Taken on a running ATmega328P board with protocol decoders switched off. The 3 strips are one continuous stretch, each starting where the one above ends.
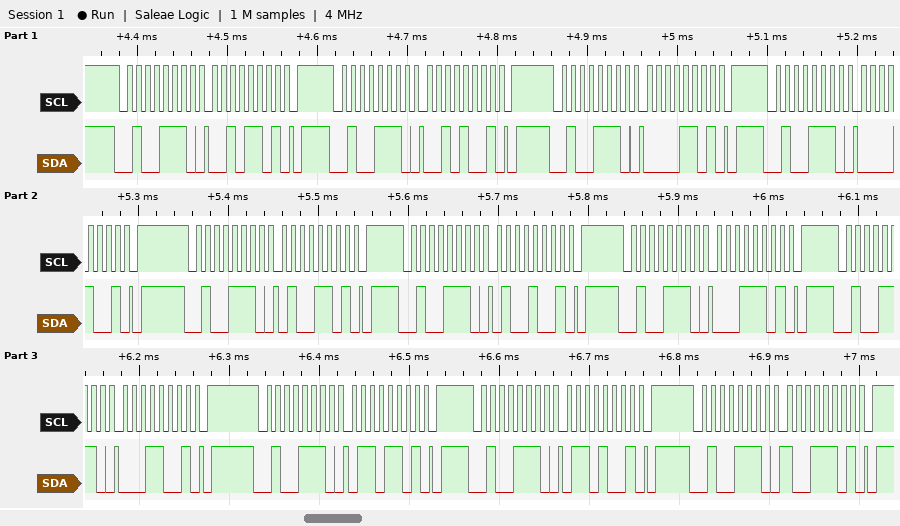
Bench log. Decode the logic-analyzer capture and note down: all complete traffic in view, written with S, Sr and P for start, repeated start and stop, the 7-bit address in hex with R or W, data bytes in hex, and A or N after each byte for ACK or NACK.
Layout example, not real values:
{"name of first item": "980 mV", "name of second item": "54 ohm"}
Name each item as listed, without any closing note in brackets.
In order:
{"all complete traffic in view, written with S, Sr and P for start, repeated start and stop, the 7-bit address in hex with R or W, data bytes in hex, and A or N after each byte for ACK or NACK": "S 27W A 2D A P S 27W A 29 A P S 27W A 0D A P S 27W A 09 A P S 27W A 4D A P S 27W A 49 A P S 27W A 1D A P S 27W A 19 A P S 27W A 6D A P S 27W A 69 A P S 27W A 9D A P"}
